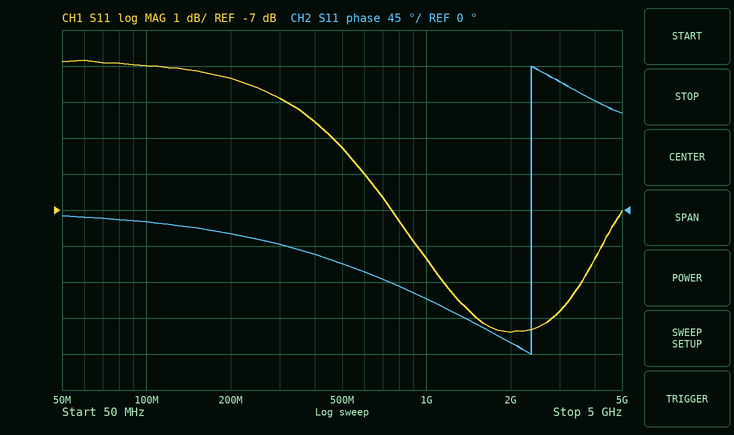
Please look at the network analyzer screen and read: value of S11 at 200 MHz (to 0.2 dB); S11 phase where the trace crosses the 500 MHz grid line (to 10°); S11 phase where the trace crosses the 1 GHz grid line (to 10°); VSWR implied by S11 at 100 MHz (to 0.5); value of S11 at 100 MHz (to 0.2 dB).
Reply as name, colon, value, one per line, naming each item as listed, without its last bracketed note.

value of S11 at 200 MHz: -3.4 dB
S11 phase where the trace crosses the 500 MHz grid line: -70°
S11 phase where the trace crosses the 1 GHz grid line: -110°
VSWR implied by S11 at 100 MHz: 6.0
value of S11 at 100 MHz: -3.0 dB
